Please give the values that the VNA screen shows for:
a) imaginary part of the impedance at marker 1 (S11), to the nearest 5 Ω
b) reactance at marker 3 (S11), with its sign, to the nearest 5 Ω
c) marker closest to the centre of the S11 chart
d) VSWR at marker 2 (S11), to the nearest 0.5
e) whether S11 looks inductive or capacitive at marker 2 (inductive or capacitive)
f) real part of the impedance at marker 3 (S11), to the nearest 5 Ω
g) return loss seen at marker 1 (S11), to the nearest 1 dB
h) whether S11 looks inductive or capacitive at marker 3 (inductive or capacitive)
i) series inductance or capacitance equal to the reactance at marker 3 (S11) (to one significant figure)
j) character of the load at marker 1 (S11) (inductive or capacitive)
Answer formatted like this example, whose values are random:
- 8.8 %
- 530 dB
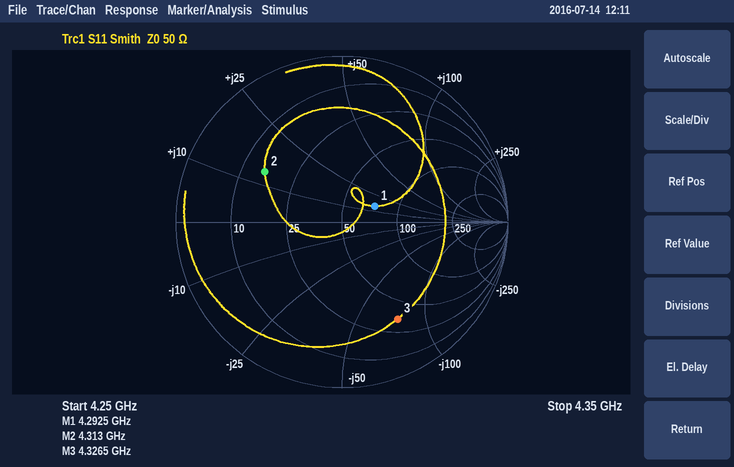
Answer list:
- +15 Ω
- -75 Ω
- marker 1
- 3.5
- inductive
- 35 Ω
- 13 dB
- capacitive
- 500 fF
- inductive
